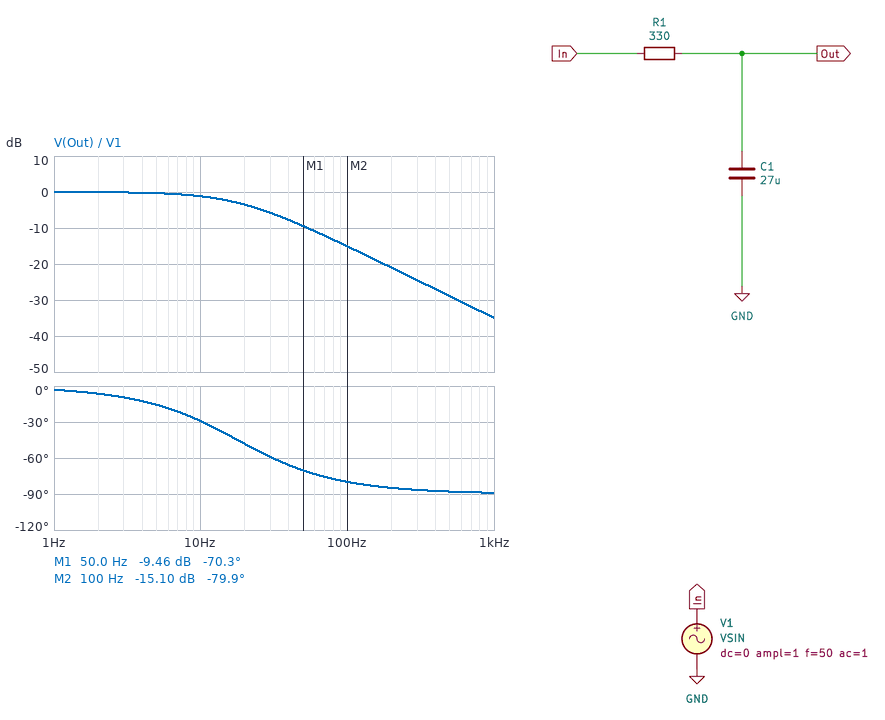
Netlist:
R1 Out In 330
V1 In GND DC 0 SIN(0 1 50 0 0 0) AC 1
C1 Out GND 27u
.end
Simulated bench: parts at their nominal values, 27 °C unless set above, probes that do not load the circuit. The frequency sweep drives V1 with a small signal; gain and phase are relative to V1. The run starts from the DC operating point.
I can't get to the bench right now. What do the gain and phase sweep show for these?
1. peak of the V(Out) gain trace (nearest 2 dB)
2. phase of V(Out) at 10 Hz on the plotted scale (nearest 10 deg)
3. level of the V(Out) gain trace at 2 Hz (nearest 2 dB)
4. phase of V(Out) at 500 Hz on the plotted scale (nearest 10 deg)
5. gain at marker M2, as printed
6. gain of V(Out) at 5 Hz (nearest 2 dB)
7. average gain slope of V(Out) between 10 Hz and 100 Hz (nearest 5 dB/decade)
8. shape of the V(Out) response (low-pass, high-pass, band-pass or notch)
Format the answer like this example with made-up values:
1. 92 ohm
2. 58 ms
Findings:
1. 0 dB
2. -30 deg
3. 0 dB
4. -90 deg
5. -15.10 dB
6. 0 dB
7. -15 dB/decade
8. low-pass
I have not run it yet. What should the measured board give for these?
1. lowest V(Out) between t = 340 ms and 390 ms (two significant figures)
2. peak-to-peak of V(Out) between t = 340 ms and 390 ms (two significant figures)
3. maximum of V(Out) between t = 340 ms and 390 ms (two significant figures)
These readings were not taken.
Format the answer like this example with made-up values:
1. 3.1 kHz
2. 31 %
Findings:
1. -340 mV
2. 670 mV
3. 340 mV
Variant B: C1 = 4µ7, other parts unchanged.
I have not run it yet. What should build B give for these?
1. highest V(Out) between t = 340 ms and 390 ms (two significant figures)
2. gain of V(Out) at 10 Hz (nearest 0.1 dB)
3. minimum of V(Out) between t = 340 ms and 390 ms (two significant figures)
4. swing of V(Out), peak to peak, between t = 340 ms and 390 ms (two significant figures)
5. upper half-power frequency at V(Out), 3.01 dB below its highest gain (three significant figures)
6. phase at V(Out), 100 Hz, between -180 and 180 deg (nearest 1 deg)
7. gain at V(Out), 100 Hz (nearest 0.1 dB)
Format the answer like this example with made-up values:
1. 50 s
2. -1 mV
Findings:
1. 900 mV
2. 0 dB
3. -900 mV
4. 1.8 V
5. 103 Hz
6. -44 deg
7. -2.9 dB
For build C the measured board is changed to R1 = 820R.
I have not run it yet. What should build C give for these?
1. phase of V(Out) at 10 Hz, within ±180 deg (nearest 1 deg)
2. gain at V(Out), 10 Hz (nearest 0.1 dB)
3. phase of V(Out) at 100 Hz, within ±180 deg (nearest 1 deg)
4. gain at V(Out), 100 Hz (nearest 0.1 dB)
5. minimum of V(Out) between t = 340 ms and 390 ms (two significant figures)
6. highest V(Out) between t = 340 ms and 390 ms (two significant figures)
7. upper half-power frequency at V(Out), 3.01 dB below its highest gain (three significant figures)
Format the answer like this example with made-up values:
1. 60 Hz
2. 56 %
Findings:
1. -54 deg
2. -4.7 dB
3. -86 deg
4. -22.9 dB
5. -140 mV
6. 140 mV
7. 7.19 Hz
